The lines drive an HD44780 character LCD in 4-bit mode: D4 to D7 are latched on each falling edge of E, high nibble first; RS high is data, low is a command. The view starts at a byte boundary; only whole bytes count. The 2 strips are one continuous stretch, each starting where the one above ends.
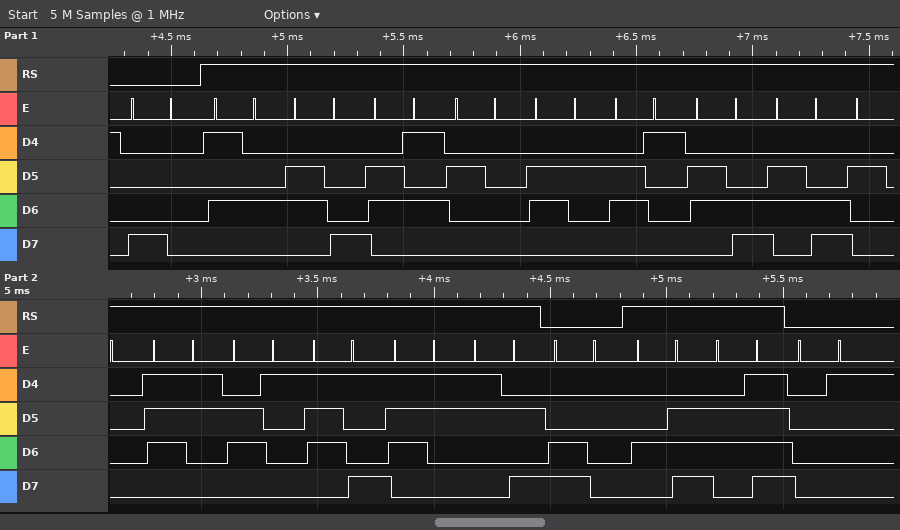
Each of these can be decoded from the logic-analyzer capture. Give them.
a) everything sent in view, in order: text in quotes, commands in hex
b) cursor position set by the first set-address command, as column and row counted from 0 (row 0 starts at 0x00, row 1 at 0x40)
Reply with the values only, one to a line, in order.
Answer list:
0x80 "The ball says:" 0xC0 "No" 0x01
column 0, row 0
